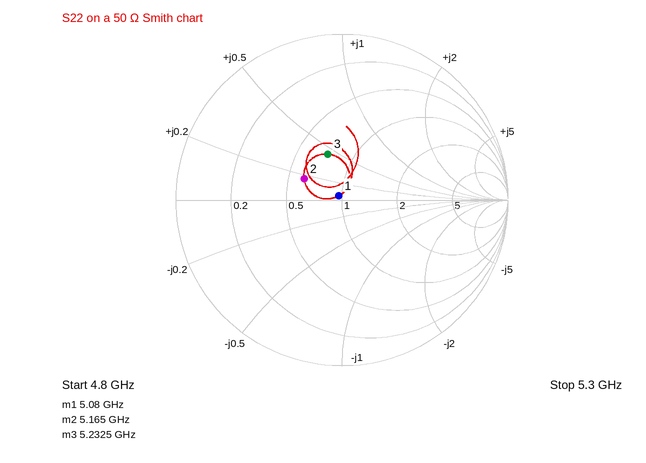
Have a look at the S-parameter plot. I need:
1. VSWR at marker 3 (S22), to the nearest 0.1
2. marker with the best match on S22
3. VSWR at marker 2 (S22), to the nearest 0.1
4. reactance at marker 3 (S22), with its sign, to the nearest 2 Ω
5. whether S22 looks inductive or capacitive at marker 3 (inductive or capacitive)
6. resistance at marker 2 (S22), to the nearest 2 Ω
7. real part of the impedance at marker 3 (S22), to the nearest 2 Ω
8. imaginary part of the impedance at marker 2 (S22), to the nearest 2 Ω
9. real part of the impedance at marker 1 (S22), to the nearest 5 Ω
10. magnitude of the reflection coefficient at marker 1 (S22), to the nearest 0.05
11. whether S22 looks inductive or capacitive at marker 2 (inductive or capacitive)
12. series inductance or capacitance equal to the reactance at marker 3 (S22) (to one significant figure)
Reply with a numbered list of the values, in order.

1. 1.8
2. marker 1
3. 1.7
4. +22 Ω
5. inductive
6. 30 Ω
7. 36 Ω
8. +8 Ω
9. 50 Ω
10. 0.05
11. inductive
12. 700 pH
